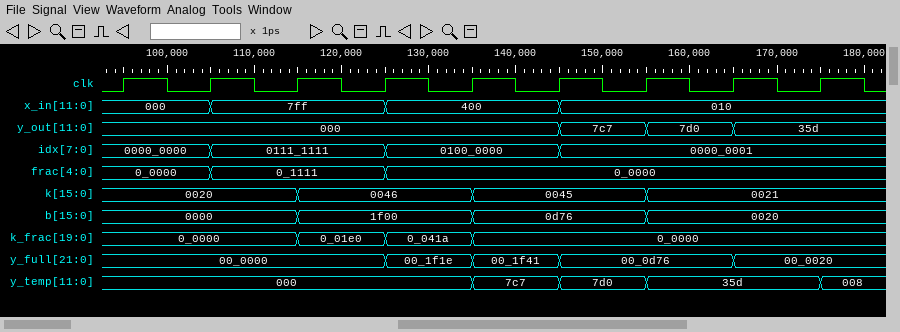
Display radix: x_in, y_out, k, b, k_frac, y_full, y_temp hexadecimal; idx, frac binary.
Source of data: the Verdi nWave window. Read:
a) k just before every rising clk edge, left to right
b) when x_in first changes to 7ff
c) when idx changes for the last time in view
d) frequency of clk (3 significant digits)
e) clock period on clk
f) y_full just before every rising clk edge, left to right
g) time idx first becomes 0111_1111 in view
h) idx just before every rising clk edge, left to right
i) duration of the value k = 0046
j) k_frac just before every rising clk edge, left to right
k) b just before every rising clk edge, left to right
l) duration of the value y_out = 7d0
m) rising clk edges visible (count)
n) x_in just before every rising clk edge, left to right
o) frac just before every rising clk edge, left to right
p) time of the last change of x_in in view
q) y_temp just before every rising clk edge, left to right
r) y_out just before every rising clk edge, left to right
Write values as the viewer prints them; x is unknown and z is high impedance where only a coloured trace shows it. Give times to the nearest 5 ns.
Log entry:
0020, 0020, 0020, 0046, 0046, 0045, 0045, 0021, 0021
105 ns
145 ns
100 MHz
10 ns
00_0000, 00_0000, 00_0000, 00_0000, 00_1f1e, 00_1f41, 00_0d76, 00_0d76, 00_0020
105 ns
0000_0000, 0000_0000, 0111_1111, 0111_1111, 0100_0000, 0100_0000, 0000_0001, 0000_0001, 0000_0001
20 ns
0_0000, 0_0000, 0_0000, 0_01e0, 0_041a, 0_0000, 0_0000, 0_0000, 0_0000
0000, 0000, 0000, 1f00, 1f00, 0d76, 0d76, 0020, 0020
10 ns
9
000, 000, 7ff, 7ff, 400, 400, 010, 010, 010
0_0000, 0_0000, 0_1111, 0_1111, 0_0000, 0_0000, 0_0000, 0_0000, 0_0000
145 ns
000, 000, 000, 000, 000, 7c7, 7d0, 35d, 35d
000, 000, 000, 000, 000, 000, 7c7, 7d0, 35d
